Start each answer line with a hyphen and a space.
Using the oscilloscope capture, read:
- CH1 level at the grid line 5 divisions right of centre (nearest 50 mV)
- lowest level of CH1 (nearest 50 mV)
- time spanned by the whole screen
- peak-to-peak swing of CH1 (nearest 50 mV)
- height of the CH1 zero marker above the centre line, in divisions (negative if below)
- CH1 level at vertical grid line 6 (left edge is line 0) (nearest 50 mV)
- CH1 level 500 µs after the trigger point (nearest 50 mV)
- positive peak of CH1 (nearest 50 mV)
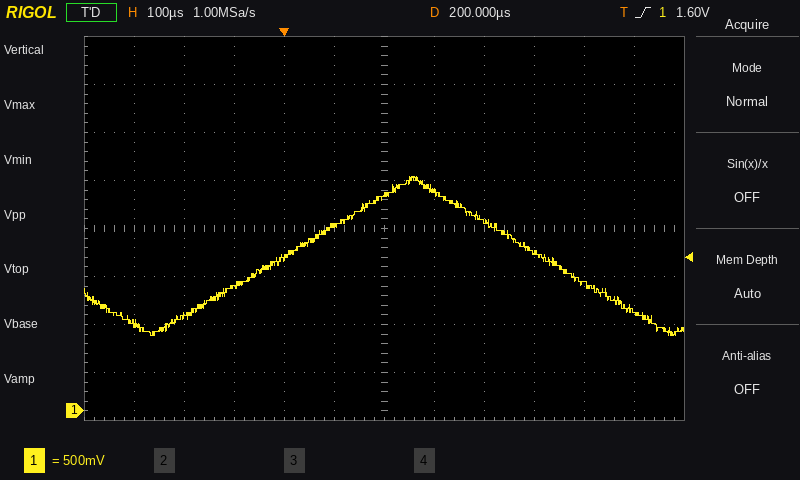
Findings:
- 1.05 V
- 800 mV
- 1.2 ms
- 1.65 V
- -3.8 div
- 2.25 V
- 1.65 V
- 2.45 V
